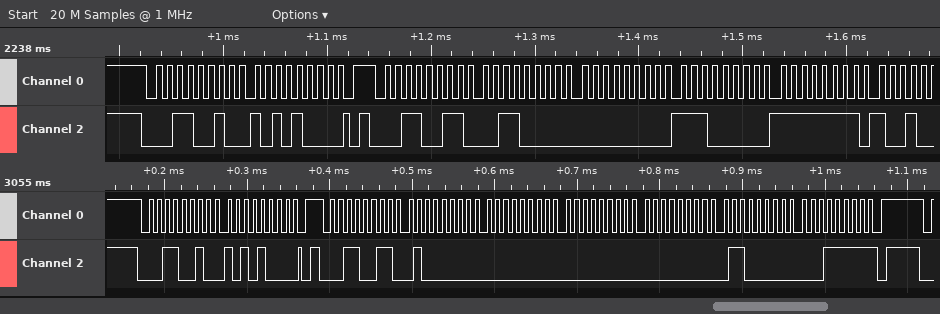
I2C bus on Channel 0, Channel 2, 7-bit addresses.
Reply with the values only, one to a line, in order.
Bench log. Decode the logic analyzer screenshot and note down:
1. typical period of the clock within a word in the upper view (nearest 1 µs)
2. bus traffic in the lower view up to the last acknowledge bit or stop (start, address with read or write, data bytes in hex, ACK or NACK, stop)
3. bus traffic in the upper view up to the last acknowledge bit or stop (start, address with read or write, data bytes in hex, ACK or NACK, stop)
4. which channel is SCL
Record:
10 µs
start, address 19 write ACK, A8 ACK, stop, start, address 19 read ACK, 40 ACK, 00 ACK, 00 ACK, 00 ACK, 60 ACK, 1F NACK, stop
start, address 19 write ACK, A8 ACK, stop, start, address 19 read ACK, 30 ACK, 00 ACK, E0 ACK, FF ACK
Channel 0
